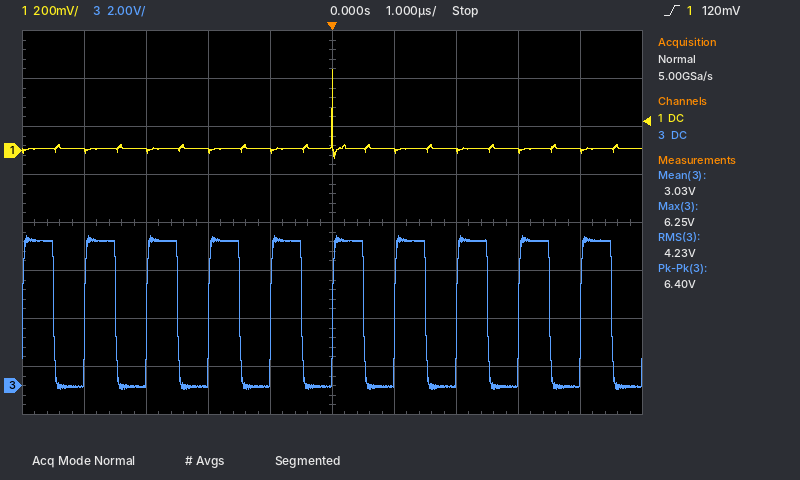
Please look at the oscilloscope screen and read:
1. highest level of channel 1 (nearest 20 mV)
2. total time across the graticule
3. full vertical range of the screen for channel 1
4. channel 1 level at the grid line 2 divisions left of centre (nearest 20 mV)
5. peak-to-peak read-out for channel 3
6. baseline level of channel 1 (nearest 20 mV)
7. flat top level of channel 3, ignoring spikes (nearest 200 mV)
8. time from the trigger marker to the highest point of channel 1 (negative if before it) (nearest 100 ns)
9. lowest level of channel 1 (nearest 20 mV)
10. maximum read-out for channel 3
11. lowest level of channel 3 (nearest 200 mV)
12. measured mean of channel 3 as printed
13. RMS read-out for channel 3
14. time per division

340 mV
10 µs
1.6 V
0 mV
6.40 V
0 mV
6.0 V
0.0 µs
-40 mV
6.25 V
-200 mV
3.03 V
4.23 V
1 µs
